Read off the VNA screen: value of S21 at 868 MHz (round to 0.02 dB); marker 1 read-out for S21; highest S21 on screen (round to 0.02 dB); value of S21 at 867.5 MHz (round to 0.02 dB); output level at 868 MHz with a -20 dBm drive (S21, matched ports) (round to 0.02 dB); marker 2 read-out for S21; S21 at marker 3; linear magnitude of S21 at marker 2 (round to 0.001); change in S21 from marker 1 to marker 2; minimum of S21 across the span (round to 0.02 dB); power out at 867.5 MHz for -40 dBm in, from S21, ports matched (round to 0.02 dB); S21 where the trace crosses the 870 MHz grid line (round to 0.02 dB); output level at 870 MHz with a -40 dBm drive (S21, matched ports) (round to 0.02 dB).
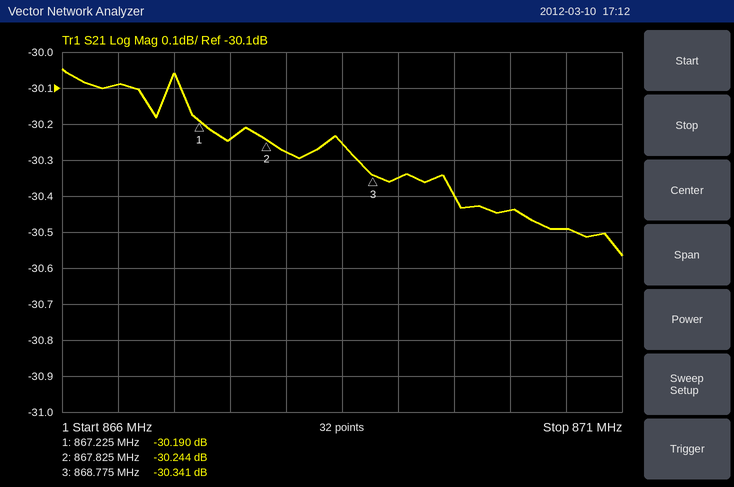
-30.28 dB
-30.190 dB
-30.04 dB
-30.24 dB
-50.28 dBm
-30.244 dB
-30.341 dB
0.031
-0.054 dB
-30.56 dB
-70.24 dBm
-30.44 dB
-70.44 dBm
